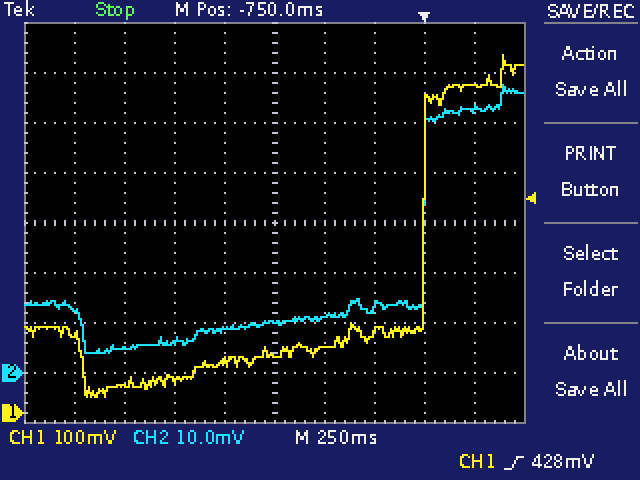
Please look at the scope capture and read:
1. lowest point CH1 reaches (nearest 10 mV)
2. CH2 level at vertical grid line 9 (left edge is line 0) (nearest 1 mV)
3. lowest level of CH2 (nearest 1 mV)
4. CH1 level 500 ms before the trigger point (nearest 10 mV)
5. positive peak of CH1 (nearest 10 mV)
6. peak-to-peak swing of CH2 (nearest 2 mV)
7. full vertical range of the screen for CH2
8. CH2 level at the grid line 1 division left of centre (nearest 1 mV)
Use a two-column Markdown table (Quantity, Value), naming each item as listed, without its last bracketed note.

| Quantity | Value |
|---|---|
| lowest point CH1 reaches | 30 mV |
| CH2 level at vertical grid line 9 (left edge is line 0) | 53 mV |
| lowest level of CH2 | 4 mV |
| CH1 level 500 ms before the trigger point | 130 mV |
| positive peak of CH1 | 720 mV |
| peak-to-peak swing of CH2 | 54 mV |
| full vertical range of the screen for CH2 | 80 mV |
| CH2 level at the grid line 1 division left of centre | 9 mV |
